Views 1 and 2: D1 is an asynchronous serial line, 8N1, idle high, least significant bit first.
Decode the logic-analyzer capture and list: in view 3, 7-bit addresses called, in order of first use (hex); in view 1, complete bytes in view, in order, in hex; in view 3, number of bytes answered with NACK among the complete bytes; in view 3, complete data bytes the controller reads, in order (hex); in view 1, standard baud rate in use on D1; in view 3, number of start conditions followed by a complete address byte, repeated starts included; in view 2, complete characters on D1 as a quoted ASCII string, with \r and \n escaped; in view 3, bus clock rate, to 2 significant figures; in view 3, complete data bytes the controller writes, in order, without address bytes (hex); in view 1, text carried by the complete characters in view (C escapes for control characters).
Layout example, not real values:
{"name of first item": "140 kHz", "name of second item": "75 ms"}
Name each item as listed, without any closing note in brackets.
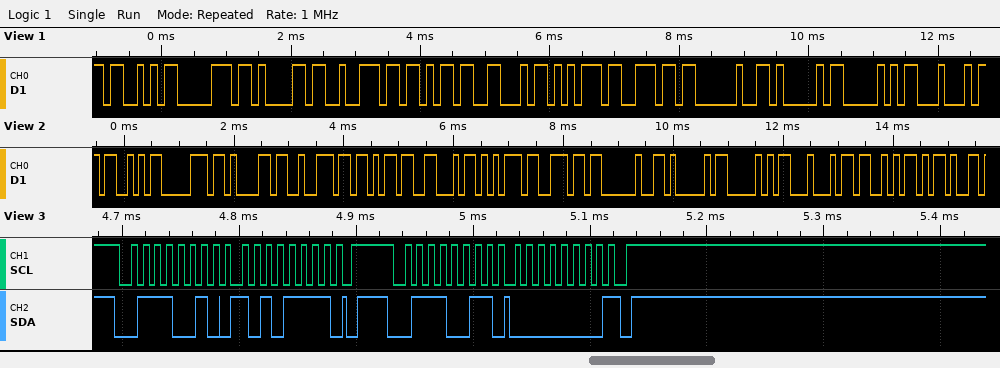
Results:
{"in view 3, 7-bit addresses called, in order of first use": "0x39", "in view 1, complete bytes in view, in order, in hex": "53 70 61 72 6B 46 75 6E 20 41 50 44", "in view 3, number of bytes answered with NACK among the complete bytes": "1", "in view 3, complete data bytes the controller reads, in order": "00", "in view 1, standard baud rate in use on D1": "9600 baud", "in view 3, number of start conditions followed by a complete address byte, repeated starts included": "2", "in view 2, complete characters on D1 as a quoted ASCII string, with \\r and \\n escaped": "\"SparkFun APDS-\"", "in view 3, bus clock rate, to 2 significant figures": "100 kHz", "in view 3, complete data bytes the controller writes, in order, without address bytes": "AF", "in view 1, text carried by the complete characters in view": "\"SparkFun APD\""}
